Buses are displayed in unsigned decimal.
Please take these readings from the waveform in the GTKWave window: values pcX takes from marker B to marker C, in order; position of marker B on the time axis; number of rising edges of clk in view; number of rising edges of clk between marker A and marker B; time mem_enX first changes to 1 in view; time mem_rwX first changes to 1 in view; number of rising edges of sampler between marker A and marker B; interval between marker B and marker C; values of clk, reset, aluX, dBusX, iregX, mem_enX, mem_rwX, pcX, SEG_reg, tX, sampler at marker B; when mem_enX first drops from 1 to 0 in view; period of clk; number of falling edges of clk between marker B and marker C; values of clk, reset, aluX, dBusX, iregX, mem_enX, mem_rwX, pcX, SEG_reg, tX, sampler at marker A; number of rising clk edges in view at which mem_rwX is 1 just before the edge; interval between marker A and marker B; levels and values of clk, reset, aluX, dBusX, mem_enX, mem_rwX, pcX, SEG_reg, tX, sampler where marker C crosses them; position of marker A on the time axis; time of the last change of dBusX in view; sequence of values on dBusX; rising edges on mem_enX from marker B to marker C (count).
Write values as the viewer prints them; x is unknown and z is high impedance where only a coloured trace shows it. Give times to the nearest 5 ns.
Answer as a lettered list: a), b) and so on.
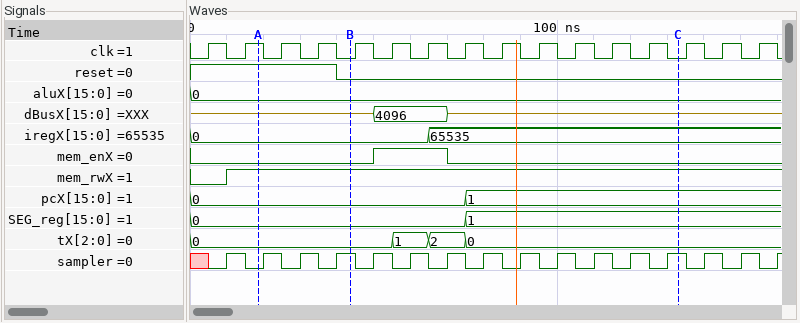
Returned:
a) 0, 1
b) 45 ns
c) 16
d) 2
e) 50 ns
f) 10 ns
g) 3
h) 90 ns
i) clk=0, reset=0, aluX=0, dBusX=z, iregX=0, mem_enX=0, mem_rwX=1, pcX=0, SEG_reg=0, tX=0, sampler=1
j) 70 ns
k) 10 ns
l) 9
m) clk=1, reset=1, aluX=0, dBusX=z, iregX=0, mem_enX=0, mem_rwX=1, pcX=0, SEG_reg=0, tX=0, sampler=0
n) 15
o) 25 ns
p) clk=0, reset=0, aluX=0, dBusX=z, mem_enX=0, mem_rwX=1, pcX=1, SEG_reg=1, tX=0, sampler=1
q) 20 ns
r) 70 ns
s) z, 4096, z
t) 1
